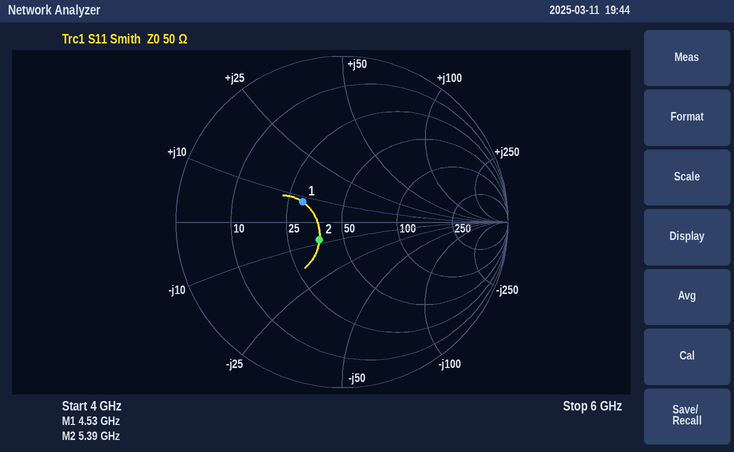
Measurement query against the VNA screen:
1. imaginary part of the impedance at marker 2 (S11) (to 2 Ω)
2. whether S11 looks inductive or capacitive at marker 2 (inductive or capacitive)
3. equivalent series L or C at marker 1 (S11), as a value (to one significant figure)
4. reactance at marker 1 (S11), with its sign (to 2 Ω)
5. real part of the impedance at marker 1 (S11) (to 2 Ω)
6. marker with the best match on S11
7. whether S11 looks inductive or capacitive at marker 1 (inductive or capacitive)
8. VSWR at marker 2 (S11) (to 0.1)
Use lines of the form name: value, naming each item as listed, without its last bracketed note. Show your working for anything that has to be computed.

imaginary part of the impedance at marker 2 (S11): -8 Ω
whether S11 looks inductive or capacitive at marker 2: capacitive
equivalent series L or C at marker 1 (S11), as a value: L = 8 Ω/(2π × 4.53 GHz) ≈ 281 pH, so 300 pH to one significant figure
reactance at marker 1 (S11), with its sign: +8 Ω
real part of the impedance at marker 1 (S11): 30 Ω
marker with the best match on S11: marker 2
whether S11 looks inductive or capacitive at marker 1: inductive
VSWR at marker 2 (S11): 1.4
